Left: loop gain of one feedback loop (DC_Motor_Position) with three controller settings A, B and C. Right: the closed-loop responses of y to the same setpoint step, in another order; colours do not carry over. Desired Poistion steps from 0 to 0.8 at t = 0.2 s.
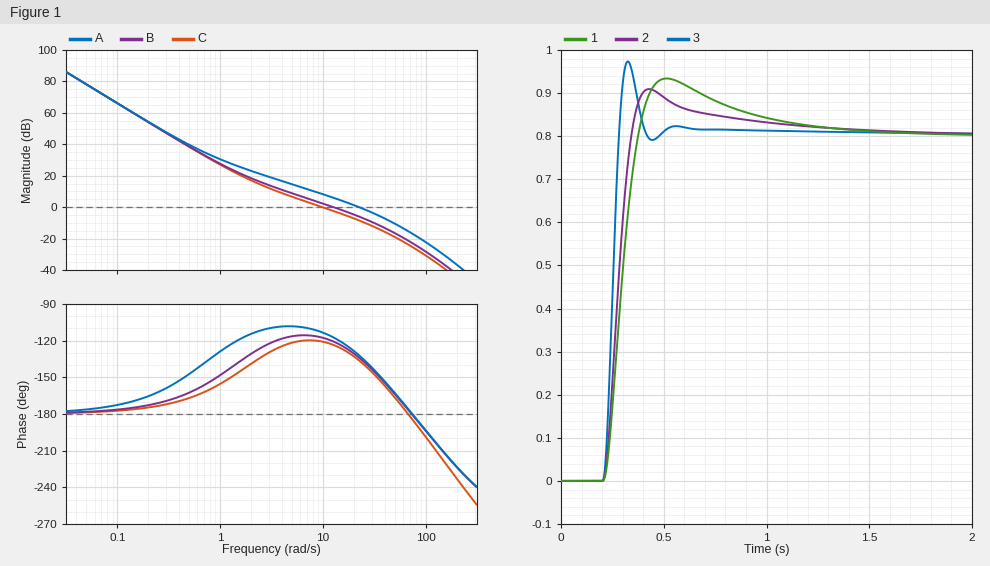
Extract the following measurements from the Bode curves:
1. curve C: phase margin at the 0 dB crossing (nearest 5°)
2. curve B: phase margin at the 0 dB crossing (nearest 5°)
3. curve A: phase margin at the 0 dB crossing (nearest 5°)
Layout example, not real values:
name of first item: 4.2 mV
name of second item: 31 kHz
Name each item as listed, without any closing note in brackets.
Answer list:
curve C: phase margin at the 0 dB crossing: 60°
curve B: phase margin at the 0 dB crossing: 60°
curve A: phase margin at the 0 dB crossing: 50°
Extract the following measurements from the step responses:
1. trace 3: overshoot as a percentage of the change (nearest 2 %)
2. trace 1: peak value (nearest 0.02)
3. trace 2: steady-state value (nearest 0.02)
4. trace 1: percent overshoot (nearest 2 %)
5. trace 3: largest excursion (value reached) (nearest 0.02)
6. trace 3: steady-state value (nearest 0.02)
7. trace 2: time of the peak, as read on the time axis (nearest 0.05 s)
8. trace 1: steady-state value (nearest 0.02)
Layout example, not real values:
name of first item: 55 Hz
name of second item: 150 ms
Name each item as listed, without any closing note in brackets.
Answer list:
trace 3: overshoot as a percentage of the change: 22 %
trace 1: peak value: 0.94
trace 2: steady-state value: 0.80
trace 1: percent overshoot: 16 %
trace 3: largest excursion (value reached): 0.98
trace 3: steady-state value: 0.80
trace 2: time of the peak, as read on the time axis: 0.45 s
trace 1: steady-state value: 0.80
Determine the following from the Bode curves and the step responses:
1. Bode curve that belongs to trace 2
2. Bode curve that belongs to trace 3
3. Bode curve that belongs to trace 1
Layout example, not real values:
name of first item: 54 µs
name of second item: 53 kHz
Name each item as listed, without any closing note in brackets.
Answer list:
Bode curve that belongs to trace 2: B
Bode curve that belongs to trace 3: A
Bode curve that belongs to trace 1: C
